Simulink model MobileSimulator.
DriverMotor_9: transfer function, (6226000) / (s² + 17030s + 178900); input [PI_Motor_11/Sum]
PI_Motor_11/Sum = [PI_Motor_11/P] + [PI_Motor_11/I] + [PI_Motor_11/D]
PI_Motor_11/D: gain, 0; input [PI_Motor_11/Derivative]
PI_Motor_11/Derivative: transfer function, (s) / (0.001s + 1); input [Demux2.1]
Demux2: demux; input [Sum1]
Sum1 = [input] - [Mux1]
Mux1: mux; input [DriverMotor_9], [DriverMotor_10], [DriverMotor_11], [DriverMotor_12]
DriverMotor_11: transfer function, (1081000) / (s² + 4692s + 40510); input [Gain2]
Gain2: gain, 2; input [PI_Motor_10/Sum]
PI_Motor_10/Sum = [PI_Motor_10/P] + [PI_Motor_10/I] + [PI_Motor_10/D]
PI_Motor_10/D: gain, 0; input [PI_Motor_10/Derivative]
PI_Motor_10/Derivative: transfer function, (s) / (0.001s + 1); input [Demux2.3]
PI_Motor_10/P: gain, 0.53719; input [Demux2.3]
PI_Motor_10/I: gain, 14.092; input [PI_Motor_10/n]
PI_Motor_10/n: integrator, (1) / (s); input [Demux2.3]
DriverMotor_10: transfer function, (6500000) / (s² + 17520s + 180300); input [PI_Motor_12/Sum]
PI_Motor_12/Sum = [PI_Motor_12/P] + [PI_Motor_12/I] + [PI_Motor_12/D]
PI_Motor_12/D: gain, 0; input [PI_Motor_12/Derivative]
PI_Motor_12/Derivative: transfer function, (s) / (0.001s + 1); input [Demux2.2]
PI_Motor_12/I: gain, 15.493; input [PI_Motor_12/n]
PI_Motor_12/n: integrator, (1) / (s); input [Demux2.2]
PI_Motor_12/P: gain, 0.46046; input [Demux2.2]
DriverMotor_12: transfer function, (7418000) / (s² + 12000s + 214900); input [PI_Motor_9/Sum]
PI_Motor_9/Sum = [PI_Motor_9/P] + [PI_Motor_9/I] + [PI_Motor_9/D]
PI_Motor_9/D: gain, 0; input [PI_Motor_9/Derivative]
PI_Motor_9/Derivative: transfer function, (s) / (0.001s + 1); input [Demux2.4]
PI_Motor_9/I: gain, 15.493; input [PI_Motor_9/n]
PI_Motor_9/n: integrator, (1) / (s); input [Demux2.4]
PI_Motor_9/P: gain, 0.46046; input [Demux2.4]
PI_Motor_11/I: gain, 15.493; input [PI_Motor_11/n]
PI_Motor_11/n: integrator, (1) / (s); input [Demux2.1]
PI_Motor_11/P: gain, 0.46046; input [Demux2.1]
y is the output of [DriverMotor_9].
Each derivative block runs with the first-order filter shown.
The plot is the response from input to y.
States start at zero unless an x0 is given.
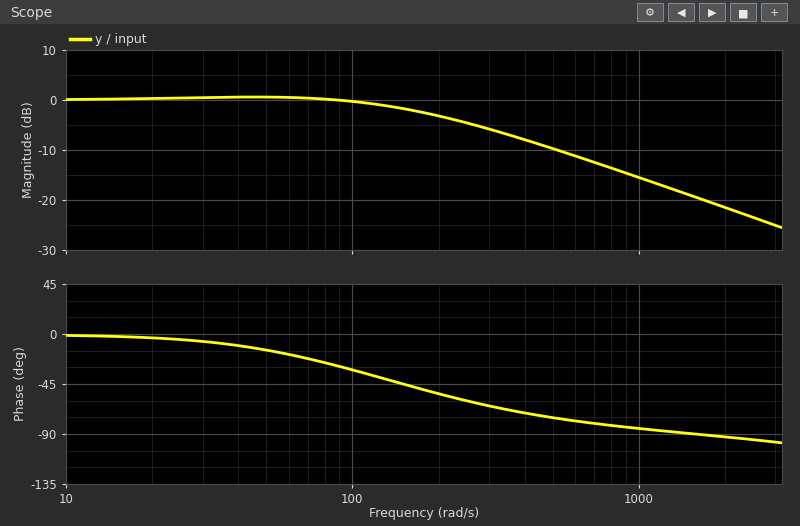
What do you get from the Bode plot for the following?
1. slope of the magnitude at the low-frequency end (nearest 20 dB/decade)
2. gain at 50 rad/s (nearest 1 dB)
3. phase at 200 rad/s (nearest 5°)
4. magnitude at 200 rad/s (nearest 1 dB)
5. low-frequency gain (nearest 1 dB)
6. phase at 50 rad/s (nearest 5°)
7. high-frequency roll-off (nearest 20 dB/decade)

0 dB/decade
1 dB
-55°
-3 dB
0 dB
-15°
-20 dB/decade
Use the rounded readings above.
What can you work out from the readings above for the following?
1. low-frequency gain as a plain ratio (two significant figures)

1.0
